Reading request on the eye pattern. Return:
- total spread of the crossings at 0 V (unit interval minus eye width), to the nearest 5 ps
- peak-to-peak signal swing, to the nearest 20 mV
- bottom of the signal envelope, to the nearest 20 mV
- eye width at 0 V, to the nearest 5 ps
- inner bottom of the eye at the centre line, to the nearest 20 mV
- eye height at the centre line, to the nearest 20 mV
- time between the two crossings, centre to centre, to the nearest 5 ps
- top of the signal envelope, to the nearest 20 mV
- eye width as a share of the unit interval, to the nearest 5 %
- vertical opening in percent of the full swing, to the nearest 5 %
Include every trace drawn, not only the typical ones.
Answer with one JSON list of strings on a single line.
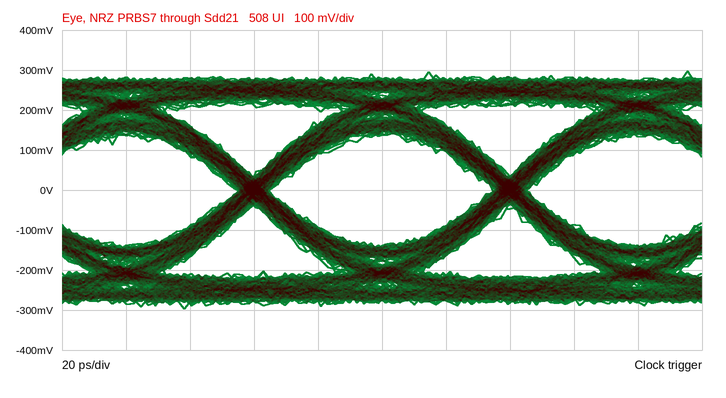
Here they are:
["10 ps", "600 mV", "-300 mV", "70 ps", "-140 mV", "280 mV", "80 ps", "300 mV", "85 %", "45 %"]
